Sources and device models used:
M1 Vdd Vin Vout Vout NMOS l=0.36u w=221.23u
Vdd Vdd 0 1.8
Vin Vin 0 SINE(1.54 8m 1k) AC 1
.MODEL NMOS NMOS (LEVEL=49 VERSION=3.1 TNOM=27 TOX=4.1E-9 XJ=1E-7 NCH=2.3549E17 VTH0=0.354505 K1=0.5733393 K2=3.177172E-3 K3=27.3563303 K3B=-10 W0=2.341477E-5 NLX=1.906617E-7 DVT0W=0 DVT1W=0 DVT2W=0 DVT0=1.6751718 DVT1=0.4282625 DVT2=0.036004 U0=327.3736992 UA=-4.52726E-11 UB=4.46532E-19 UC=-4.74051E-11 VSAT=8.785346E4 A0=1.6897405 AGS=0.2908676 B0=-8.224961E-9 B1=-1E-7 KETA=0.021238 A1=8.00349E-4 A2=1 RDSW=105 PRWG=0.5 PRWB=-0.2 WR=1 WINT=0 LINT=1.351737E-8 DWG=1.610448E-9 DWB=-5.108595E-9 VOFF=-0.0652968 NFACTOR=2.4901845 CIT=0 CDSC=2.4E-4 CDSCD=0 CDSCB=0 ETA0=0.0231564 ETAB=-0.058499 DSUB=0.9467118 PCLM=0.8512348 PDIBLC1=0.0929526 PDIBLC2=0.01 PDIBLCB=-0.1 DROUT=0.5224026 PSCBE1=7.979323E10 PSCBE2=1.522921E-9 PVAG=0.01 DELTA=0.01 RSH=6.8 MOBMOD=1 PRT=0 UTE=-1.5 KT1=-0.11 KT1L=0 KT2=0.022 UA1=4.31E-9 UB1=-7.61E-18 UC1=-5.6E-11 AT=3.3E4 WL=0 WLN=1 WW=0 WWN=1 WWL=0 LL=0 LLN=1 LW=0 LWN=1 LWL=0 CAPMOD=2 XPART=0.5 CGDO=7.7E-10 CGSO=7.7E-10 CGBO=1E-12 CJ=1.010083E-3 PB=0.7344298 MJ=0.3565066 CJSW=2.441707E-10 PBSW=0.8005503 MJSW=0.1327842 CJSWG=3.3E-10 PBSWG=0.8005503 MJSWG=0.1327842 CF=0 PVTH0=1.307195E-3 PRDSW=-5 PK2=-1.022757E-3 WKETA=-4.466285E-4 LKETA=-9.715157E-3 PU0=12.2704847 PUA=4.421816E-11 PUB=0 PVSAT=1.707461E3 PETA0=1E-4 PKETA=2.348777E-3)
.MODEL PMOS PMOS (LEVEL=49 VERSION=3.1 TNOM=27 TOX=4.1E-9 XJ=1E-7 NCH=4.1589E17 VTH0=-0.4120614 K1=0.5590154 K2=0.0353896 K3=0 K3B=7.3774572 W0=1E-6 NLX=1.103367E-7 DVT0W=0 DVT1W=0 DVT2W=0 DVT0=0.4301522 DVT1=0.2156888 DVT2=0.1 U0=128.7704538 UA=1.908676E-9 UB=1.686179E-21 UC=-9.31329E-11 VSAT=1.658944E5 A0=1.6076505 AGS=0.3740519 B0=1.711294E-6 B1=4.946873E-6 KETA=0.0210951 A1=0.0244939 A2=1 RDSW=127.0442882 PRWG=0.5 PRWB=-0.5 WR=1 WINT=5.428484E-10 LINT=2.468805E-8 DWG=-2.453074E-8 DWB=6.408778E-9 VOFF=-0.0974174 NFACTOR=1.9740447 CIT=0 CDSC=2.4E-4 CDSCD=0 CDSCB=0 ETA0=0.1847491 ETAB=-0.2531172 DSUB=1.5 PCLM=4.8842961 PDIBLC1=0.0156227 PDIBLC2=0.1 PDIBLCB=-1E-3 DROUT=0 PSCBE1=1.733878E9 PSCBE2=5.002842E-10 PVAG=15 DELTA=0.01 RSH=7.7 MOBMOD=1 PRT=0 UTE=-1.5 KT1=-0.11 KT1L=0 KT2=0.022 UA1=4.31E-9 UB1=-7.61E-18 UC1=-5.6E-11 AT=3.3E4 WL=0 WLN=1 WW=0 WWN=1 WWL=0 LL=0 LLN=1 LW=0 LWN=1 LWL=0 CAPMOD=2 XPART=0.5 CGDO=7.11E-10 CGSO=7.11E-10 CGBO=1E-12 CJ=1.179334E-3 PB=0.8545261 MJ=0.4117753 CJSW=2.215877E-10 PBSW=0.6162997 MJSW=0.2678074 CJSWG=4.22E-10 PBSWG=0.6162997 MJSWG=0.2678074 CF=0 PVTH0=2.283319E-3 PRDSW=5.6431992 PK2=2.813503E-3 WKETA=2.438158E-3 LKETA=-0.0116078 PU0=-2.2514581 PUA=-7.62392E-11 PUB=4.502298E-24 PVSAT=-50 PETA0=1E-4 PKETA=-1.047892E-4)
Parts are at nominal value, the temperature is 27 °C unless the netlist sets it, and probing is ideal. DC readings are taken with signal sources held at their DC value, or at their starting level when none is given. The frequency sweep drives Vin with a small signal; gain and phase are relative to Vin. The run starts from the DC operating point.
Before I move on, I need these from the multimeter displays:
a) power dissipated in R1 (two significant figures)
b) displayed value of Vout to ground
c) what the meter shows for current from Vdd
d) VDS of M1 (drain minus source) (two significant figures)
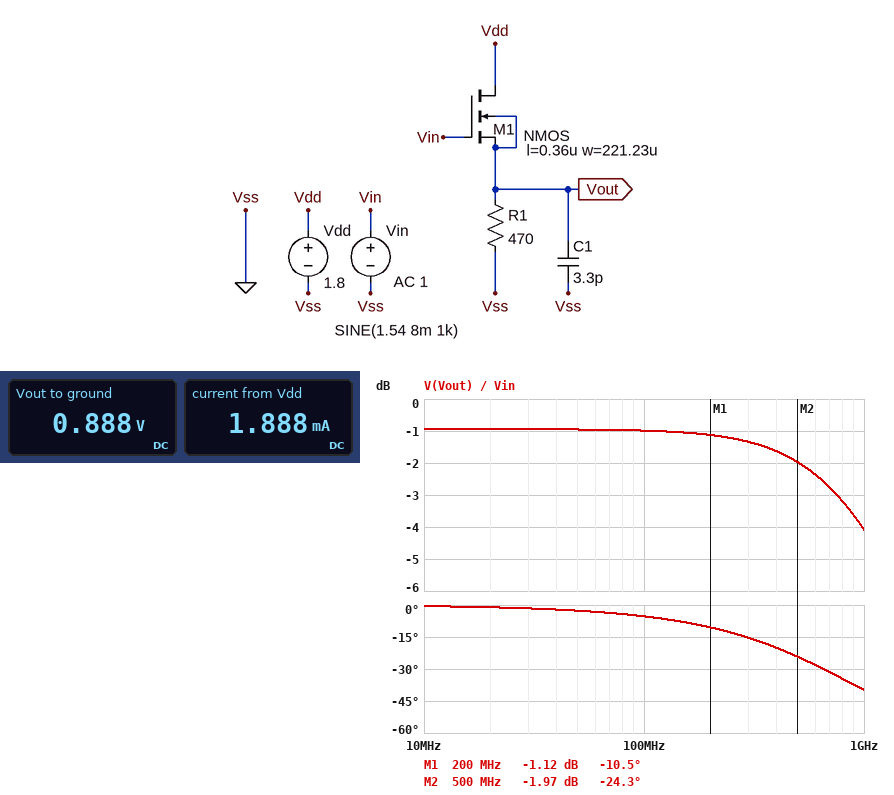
1.7 mW
0.888 V
1.888 mA
910 mV
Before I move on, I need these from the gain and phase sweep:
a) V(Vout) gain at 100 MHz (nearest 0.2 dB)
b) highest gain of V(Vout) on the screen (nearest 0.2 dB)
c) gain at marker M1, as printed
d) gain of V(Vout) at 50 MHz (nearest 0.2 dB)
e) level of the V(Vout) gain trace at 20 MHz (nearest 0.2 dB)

-1.0 dB
-1.0 dB
-1.12 dB
-1.0 dB
-1.0 dB
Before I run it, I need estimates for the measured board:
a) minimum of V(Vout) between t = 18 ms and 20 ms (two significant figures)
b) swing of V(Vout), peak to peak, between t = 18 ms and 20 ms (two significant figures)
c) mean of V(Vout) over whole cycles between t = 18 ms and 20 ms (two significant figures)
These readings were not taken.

880 mV
14 mV
890 mV
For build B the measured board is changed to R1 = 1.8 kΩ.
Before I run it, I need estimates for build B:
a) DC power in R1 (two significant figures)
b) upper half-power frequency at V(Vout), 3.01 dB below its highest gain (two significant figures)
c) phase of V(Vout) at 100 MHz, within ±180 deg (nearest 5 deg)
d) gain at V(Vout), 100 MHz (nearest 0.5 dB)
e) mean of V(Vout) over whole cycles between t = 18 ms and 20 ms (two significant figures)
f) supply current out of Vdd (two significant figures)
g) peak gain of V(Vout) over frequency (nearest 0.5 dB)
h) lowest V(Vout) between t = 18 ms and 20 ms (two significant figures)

530 µW
430 MHz
-10 deg
-1.0 dB
980 mV
540 µA
-0.5 dB
970 mV
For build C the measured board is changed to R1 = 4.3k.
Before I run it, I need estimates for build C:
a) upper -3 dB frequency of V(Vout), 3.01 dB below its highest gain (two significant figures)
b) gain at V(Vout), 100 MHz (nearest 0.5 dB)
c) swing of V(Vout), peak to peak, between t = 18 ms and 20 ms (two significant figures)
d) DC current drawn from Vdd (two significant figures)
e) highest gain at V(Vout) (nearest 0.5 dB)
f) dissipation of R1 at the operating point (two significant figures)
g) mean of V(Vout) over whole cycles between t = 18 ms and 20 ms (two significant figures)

220 MHz
-1.5 dB
15 mV
240 µA
-0.5 dB
240 µW
1.0 V
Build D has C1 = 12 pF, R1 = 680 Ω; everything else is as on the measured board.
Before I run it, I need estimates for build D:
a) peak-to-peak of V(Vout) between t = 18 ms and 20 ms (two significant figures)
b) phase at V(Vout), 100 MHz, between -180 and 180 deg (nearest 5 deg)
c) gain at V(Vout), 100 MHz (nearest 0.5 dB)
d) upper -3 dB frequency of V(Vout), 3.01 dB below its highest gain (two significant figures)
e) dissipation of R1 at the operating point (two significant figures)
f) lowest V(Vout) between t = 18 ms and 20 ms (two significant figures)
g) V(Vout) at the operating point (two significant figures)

15 mV
-20 deg
-1.5 dB
240 MHz
1.2 mW
910 mV
920 mV
